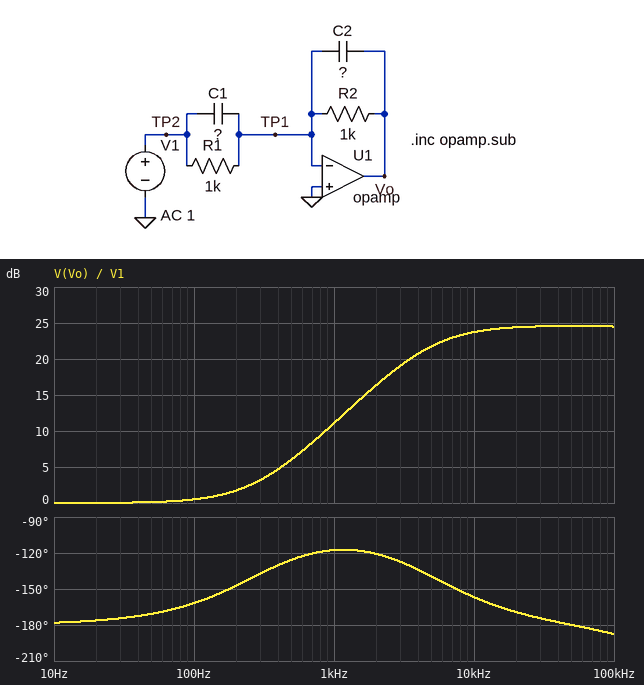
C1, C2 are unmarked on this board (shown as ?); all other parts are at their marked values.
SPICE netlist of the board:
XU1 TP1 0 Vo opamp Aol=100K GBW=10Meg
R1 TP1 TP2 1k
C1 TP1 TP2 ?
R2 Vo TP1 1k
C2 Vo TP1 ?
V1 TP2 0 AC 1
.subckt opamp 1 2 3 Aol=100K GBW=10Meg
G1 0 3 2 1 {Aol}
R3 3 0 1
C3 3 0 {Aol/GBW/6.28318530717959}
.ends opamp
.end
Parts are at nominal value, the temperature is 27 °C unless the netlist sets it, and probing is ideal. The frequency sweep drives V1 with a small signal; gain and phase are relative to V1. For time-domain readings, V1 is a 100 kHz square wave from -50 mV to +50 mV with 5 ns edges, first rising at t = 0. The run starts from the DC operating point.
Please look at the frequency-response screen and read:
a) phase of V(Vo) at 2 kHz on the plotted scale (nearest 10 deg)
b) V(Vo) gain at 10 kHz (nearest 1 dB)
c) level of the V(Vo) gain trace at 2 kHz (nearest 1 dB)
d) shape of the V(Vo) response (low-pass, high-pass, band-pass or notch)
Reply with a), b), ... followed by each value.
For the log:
a) -120 deg
b) 24 dB
c) 16 dB
d) high-pass
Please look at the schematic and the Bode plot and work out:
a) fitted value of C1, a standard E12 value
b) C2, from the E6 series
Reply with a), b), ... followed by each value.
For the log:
a) 560 nF
b) 33 nF
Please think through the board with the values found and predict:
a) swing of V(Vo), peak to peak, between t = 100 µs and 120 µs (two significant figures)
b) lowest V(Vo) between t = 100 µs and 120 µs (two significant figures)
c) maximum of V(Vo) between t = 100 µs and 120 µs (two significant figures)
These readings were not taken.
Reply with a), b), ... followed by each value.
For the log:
a) 1.8 V
b) -910 mV
c) 850 mV
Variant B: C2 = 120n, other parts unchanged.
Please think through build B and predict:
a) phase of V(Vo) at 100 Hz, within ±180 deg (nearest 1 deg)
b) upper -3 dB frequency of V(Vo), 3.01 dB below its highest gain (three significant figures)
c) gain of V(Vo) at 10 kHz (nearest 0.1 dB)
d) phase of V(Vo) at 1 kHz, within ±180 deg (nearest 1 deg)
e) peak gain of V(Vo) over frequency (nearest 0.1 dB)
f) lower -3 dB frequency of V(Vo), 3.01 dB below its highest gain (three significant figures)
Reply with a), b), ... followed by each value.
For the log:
a) -165 deg
b) 1.77 MHz
c) 13.3 dB
d) -143 deg
e) 13.4 dB
f) 1.26 kHz
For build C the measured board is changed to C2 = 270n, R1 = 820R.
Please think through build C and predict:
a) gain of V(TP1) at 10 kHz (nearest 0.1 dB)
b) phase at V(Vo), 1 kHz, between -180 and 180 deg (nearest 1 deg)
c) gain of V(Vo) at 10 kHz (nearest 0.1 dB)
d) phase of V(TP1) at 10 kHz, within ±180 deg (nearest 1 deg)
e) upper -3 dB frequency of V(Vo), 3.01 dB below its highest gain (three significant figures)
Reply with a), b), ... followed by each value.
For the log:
a) -53.7 dB
b) -169 deg
c) 6.3 dB
d) 91 deg
e) 3.25 MHz
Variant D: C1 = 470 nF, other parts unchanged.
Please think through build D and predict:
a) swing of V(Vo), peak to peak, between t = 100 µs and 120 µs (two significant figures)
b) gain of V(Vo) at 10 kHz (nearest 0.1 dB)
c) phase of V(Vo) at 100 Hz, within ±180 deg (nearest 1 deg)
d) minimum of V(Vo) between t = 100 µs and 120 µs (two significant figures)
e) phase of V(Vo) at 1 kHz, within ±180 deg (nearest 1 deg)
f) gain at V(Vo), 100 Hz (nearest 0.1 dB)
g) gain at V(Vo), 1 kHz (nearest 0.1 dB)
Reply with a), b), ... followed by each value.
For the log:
a) 1.5 V
b) 22.2 dB
c) -165 deg
d) -770 mV
e) -120 deg
f) 0.4 dB
g) 9.7 dB
